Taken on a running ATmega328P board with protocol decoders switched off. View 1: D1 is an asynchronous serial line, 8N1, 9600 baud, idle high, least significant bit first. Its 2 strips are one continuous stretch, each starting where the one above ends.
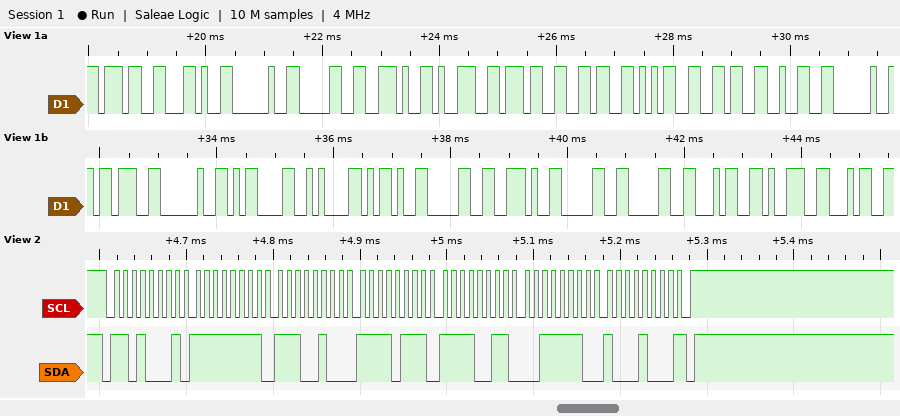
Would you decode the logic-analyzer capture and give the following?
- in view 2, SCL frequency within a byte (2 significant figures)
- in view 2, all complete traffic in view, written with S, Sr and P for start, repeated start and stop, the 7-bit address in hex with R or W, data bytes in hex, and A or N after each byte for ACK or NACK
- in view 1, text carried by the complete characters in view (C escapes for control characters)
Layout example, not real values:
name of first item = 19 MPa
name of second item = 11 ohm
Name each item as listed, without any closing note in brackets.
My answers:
in view 2, SCL frequency within a byte = 100 kHz
in view 2, all complete traffic in view, written with S, Sr and P for start, repeated start and stop, the 7-bit address in hex with R or W, data bytes in hex, and A or N after each byte for ACK or NACK = S 68R A FF A E4 A F7 A F3 A 3E A 88 N P
in view 1, text carried by the complete characters in view = "7, 0.976562 ; \r\n-0.00494"
